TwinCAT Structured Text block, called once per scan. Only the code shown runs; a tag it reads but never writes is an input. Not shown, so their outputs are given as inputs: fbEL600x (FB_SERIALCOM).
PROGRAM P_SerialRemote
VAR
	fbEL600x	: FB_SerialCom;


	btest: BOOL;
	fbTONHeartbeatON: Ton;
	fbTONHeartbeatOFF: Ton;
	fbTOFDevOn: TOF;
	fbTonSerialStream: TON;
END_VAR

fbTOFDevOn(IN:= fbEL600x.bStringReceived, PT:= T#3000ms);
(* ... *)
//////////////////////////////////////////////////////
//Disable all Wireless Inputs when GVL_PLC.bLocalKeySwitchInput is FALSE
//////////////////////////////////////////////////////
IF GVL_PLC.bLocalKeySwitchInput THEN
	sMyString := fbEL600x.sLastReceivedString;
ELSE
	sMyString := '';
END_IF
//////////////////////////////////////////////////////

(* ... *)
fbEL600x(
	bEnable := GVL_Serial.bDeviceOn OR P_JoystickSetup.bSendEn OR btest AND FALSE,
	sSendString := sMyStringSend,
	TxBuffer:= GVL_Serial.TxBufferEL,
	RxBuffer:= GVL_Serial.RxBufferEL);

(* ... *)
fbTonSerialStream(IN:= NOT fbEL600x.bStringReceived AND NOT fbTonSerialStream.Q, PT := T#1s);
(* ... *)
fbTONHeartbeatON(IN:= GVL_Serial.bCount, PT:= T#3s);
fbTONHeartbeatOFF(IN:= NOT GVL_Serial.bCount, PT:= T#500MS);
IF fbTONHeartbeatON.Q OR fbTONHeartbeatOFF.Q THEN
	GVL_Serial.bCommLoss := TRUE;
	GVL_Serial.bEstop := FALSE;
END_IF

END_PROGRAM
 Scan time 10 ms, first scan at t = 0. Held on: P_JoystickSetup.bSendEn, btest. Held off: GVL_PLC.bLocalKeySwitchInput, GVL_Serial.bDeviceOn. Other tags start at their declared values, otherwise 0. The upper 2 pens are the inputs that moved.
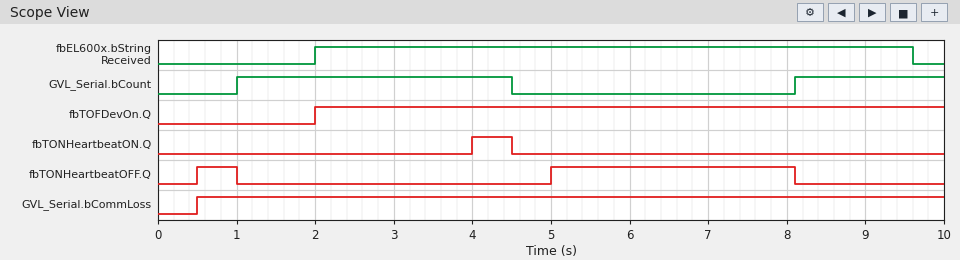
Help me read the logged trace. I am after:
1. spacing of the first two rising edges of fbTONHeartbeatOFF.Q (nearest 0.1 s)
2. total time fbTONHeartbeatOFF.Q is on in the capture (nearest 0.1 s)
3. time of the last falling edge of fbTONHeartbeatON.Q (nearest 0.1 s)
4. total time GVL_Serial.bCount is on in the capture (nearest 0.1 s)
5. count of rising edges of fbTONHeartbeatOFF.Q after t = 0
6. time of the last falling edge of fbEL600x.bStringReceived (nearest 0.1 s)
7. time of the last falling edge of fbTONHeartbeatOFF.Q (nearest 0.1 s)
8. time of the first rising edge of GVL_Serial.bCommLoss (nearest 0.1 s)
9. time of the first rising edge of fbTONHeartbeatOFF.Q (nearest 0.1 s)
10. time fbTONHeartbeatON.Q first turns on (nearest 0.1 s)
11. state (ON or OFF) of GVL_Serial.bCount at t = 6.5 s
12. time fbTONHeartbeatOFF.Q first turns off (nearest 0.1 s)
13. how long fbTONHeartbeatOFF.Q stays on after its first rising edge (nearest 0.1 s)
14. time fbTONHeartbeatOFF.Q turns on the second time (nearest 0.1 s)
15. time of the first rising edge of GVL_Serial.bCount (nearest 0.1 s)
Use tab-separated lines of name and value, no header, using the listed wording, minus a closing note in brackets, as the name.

spacing of the first two rising edges of fbTONHeartbeatOFF.Q	4.5 s
total time fbTONHeartbeatOFF.Q is on in the capture	3.6 s
time of the last falling edge of fbTONHeartbeatON.Q	4.5 s
total time GVL_Serial.bCount is on in the capture	5.4 s
count of rising edges of fbTONHeartbeatOFF.Q after t = 0	2
time of the last falling edge of fbEL600x.bStringReceived	9.6 s
time of the last falling edge of fbTONHeartbeatOFF.Q	8.1 s
time of the first rising edge of GVL_Serial.bCommLoss	0.5 s
time of the first rising edge of fbTONHeartbeatOFF.Q	0.5 s
time fbTONHeartbeatON.Q first turns on	4.0 s
state (ON or OFF) of GVL_Serial.bCount at t = 6.5 s	OFF
time fbTONHeartbeatOFF.Q first turns off	1.0 s
how long fbTONHeartbeatOFF.Q stays on after its first rising edge	0.5 s
time fbTONHeartbeatOFF.Q turns on the second time	5.0 s
time of the first rising edge of GVL_Serial.bCount	1.0 s
